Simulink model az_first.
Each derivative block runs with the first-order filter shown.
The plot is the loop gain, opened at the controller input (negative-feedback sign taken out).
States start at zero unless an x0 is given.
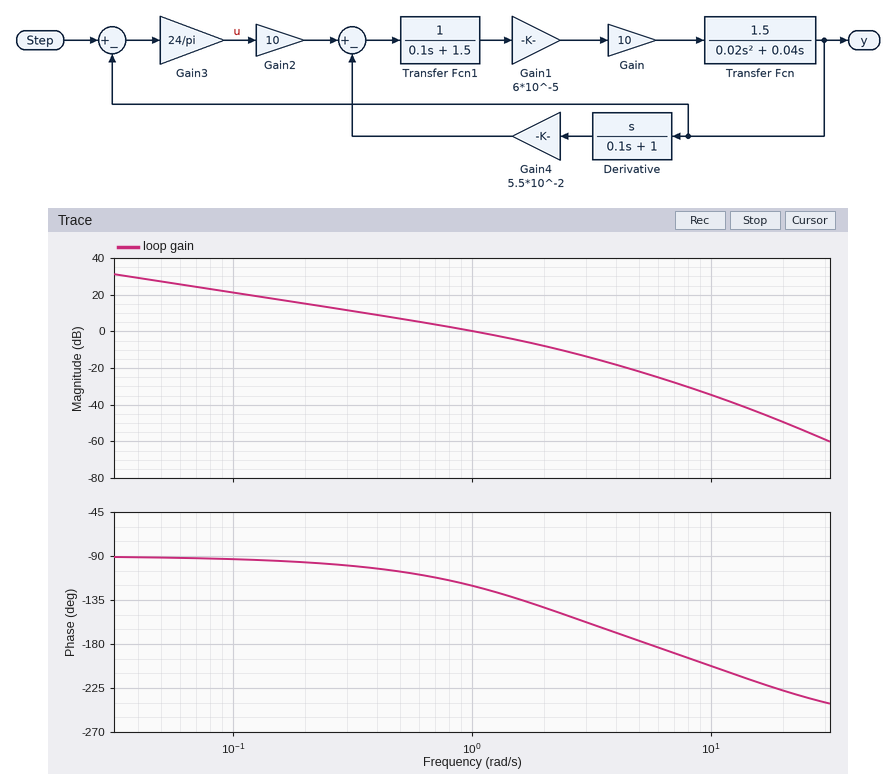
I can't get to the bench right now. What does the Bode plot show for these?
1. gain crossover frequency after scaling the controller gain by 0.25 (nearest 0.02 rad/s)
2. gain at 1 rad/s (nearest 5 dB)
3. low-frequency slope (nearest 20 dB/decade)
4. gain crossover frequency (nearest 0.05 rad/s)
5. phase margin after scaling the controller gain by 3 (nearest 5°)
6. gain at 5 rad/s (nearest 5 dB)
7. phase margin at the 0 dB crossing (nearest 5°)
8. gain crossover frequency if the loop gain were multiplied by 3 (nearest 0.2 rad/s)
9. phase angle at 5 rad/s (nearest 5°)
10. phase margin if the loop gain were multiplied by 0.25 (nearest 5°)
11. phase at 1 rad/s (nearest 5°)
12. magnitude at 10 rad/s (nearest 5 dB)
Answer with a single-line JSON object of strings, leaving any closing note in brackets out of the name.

{"gain crossover frequency after scaling the controller gain by 0.25": "0.28 rad/s", "gain at 1 rad/s": "0 dB", "low-frequency slope": "-20 dB/decade", "gain crossover frequency": "1.00 rad/s", "phase margin after scaling the controller gain by 3": "35°", "gain at 5 rad/s": "-20 dB", "phase margin at the 0 dB crossing": "60°", "gain crossover frequency if the loop gain were multiplied by 3": "2.2 rad/s", "phase angle at 5 rad/s": "-175°", "phase margin if the loop gain were multiplied by 0.25": "80°", "phase at 1 rad/s": "-120°", "magnitude at 10 rad/s": "-35 dB"}
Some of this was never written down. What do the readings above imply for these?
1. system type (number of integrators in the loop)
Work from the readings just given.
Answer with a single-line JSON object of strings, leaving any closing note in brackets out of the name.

{"system type": "1"}
